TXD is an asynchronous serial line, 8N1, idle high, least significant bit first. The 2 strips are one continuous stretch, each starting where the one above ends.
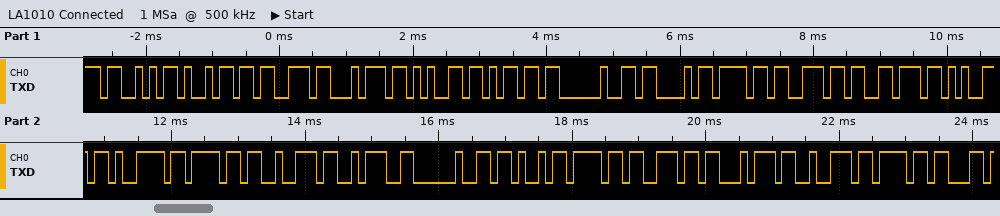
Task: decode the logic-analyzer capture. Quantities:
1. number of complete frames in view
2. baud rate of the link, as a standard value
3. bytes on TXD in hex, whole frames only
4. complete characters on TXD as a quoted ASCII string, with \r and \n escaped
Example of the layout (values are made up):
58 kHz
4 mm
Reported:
23
9600 baud
53 69 73 74 65 6D 20 43 6F 6E 76 65 79 6F 72 3A 20 4B 6F 6E 74 72 6F
"Sistem Conveyor: Kontro"
